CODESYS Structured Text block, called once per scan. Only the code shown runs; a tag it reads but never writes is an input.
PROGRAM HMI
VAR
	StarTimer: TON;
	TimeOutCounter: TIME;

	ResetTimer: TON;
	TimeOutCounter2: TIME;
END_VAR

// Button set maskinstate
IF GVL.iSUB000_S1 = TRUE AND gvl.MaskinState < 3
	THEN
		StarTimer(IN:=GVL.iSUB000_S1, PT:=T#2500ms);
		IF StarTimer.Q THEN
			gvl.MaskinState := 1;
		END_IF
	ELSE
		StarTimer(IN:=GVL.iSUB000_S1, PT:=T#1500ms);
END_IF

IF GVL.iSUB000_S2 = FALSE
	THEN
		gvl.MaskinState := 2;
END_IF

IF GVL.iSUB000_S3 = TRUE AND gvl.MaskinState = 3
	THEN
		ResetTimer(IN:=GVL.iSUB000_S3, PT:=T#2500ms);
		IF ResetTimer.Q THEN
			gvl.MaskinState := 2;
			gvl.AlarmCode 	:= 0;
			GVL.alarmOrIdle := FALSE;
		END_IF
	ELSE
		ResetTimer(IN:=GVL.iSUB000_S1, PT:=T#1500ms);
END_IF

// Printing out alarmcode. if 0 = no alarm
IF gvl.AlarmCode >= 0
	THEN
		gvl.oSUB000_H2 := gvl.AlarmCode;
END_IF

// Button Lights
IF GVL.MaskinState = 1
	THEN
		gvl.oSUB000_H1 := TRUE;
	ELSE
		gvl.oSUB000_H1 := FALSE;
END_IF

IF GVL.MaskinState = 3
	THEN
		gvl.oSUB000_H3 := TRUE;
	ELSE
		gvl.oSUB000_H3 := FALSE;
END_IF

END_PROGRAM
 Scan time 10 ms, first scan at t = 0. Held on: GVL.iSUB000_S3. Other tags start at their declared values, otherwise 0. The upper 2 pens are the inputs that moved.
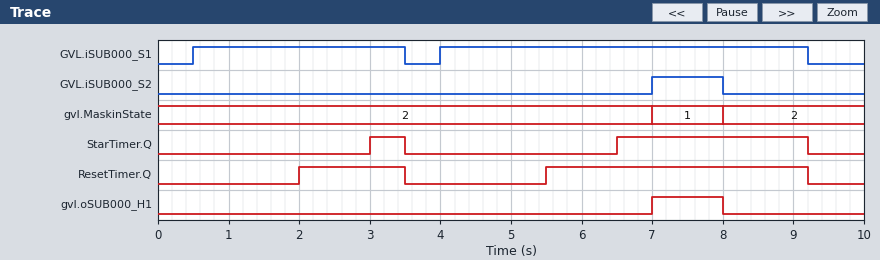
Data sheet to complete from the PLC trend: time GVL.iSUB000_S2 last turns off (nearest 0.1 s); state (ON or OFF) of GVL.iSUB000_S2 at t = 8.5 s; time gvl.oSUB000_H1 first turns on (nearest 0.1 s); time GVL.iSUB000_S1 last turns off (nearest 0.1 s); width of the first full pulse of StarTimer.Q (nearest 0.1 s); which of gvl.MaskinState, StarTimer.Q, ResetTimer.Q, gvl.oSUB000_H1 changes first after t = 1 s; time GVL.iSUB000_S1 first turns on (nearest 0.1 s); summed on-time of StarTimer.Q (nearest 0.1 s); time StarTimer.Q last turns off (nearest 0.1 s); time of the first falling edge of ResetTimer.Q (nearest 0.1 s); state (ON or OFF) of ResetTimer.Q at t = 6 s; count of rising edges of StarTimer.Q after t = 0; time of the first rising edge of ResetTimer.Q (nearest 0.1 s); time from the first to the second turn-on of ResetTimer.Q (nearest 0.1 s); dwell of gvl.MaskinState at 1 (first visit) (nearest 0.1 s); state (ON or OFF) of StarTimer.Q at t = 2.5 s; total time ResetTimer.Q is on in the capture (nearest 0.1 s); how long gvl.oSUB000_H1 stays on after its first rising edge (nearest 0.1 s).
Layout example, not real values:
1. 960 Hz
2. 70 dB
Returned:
1. 8.0 s
2. OFF
3. 7.0 s
4. 9.2 s
5. 0.5 s
6. ResetTimer.Q
7. 0.5 s
8. 3.2 s
9. 9.2 s
10. 3.5 s
11. ON
12. 2
13. 2.0 s
14. 3.5 s
15. 1.0 s
16. OFF
17. 5.2 s
18. 1.0 s
